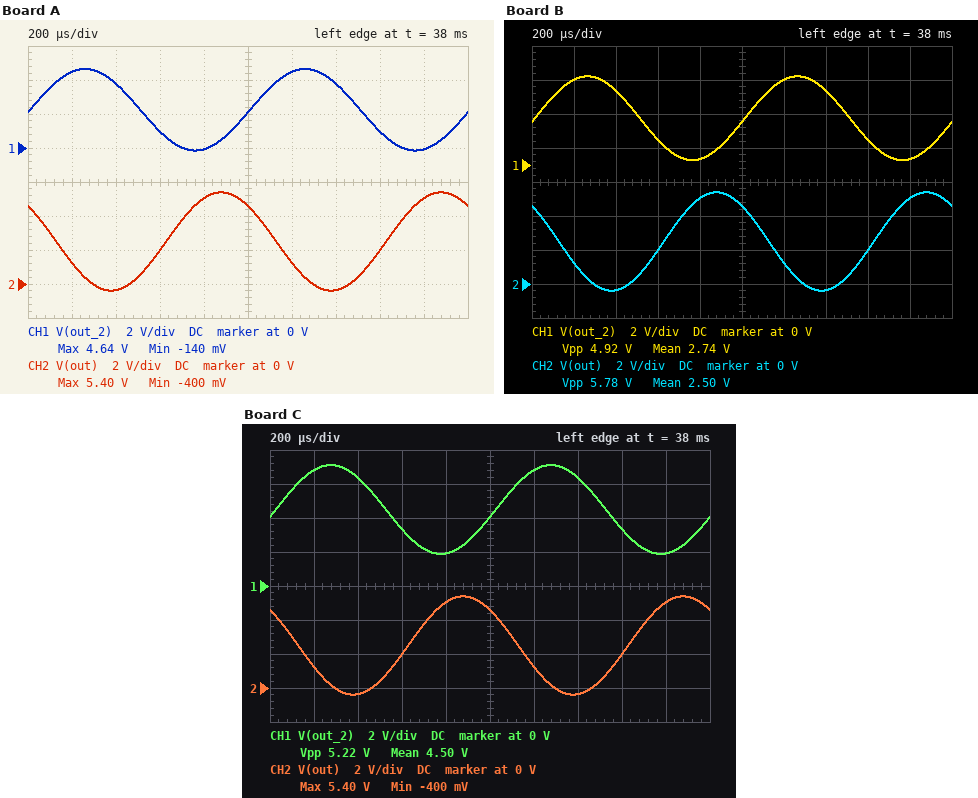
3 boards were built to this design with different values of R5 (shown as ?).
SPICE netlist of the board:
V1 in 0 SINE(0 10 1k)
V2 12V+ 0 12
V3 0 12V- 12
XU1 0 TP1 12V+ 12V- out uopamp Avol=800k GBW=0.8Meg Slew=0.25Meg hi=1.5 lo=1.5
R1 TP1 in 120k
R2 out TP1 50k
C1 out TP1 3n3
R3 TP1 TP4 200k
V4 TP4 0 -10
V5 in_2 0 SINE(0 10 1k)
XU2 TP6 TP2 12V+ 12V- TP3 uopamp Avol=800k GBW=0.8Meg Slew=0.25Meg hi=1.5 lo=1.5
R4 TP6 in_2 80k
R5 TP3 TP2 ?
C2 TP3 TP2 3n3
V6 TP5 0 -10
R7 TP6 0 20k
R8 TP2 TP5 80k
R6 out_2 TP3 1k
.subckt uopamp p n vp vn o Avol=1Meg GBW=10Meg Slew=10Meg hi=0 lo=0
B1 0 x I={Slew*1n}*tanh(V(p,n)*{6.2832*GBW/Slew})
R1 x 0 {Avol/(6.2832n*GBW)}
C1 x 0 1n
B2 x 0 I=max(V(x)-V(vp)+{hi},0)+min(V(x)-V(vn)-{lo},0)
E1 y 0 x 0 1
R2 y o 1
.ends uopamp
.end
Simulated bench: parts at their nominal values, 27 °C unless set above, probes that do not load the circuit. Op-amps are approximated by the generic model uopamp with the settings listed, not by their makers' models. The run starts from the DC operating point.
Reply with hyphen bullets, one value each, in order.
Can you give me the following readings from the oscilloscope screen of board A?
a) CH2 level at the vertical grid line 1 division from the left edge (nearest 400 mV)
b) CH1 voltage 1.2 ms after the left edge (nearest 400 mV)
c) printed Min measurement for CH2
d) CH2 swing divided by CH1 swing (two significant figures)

- 1.2 V
- 4.4 V
- -400 mV
- 1.2
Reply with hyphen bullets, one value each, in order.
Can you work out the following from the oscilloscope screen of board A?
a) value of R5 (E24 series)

- 18 kΩ
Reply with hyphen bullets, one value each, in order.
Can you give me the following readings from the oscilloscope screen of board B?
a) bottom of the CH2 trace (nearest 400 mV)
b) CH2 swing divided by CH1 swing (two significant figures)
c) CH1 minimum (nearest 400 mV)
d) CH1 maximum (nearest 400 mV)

- -400 mV
- 1.2
- 400 mV
- 5.2 V
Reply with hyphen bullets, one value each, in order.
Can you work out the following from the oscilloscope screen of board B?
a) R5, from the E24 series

- 22 kΩ
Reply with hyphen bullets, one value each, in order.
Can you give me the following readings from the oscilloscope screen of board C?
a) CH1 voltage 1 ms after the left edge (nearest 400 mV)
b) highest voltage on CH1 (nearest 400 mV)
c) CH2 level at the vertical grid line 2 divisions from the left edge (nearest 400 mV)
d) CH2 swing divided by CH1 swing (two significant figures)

- 4.0 V
- 7.2 V
- -400 mV
- 1.1
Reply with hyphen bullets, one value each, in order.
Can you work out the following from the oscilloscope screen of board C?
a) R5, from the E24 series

- 36 kΩ
